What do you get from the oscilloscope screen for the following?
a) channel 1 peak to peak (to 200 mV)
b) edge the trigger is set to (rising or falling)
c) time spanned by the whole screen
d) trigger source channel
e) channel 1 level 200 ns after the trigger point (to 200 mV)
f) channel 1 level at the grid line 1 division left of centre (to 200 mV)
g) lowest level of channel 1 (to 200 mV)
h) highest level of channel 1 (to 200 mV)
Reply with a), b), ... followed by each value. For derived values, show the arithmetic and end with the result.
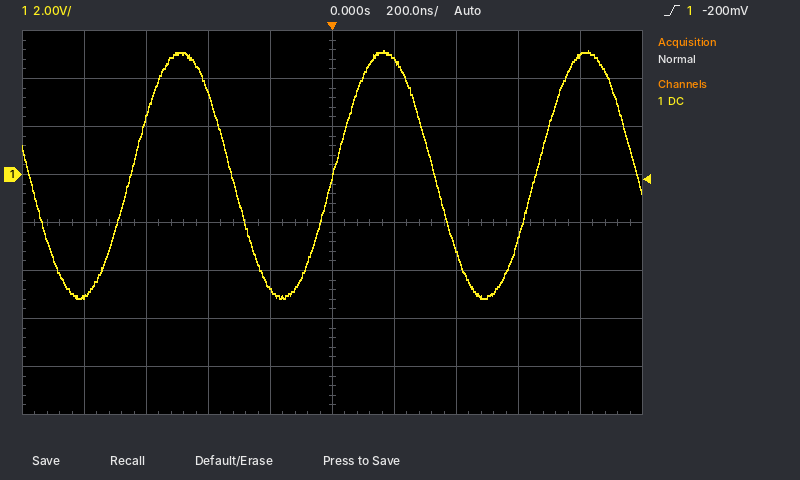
a) 5.2 V − (-5.2 V) = 10.4 V
b) rising
c) 2 µs
d) channel 1
e) 4.8 V
f) -4.8 V
g) -5.2 V
h) 5.2 V
